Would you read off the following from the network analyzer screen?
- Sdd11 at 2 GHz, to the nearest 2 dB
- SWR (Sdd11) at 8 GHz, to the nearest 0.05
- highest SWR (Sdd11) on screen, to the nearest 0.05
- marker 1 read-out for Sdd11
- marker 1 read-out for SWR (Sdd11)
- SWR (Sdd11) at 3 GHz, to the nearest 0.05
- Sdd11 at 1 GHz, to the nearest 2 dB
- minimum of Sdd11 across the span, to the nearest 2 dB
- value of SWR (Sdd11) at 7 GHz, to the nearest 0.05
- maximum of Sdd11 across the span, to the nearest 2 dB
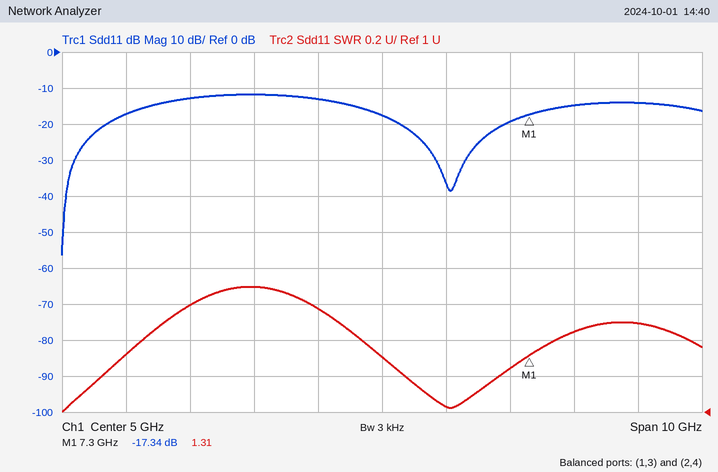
-12 dB
1.45
1.70
-17.34 dB
1.31
1.70
-18 dB
-56 dB
1.25
-12 dB
